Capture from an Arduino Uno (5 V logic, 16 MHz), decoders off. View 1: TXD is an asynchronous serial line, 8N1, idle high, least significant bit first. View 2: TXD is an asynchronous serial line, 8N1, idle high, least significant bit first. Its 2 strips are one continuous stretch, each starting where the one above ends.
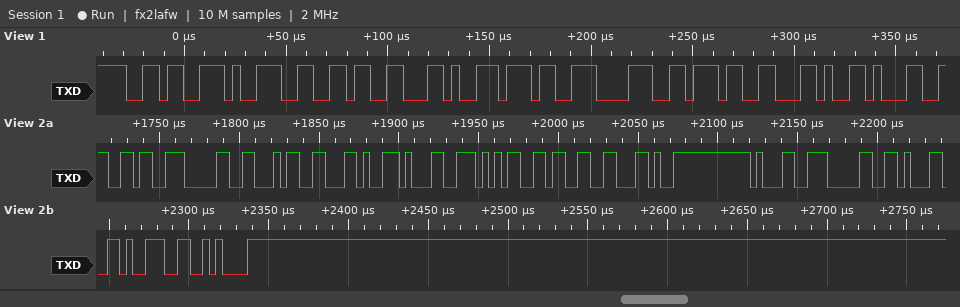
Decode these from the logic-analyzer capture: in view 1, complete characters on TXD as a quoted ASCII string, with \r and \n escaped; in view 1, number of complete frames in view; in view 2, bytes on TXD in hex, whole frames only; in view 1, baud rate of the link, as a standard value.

"696,787,1"
9
36 30 34 2C 31 35 33 2C 31 30 31 39 0A
250000 baud
